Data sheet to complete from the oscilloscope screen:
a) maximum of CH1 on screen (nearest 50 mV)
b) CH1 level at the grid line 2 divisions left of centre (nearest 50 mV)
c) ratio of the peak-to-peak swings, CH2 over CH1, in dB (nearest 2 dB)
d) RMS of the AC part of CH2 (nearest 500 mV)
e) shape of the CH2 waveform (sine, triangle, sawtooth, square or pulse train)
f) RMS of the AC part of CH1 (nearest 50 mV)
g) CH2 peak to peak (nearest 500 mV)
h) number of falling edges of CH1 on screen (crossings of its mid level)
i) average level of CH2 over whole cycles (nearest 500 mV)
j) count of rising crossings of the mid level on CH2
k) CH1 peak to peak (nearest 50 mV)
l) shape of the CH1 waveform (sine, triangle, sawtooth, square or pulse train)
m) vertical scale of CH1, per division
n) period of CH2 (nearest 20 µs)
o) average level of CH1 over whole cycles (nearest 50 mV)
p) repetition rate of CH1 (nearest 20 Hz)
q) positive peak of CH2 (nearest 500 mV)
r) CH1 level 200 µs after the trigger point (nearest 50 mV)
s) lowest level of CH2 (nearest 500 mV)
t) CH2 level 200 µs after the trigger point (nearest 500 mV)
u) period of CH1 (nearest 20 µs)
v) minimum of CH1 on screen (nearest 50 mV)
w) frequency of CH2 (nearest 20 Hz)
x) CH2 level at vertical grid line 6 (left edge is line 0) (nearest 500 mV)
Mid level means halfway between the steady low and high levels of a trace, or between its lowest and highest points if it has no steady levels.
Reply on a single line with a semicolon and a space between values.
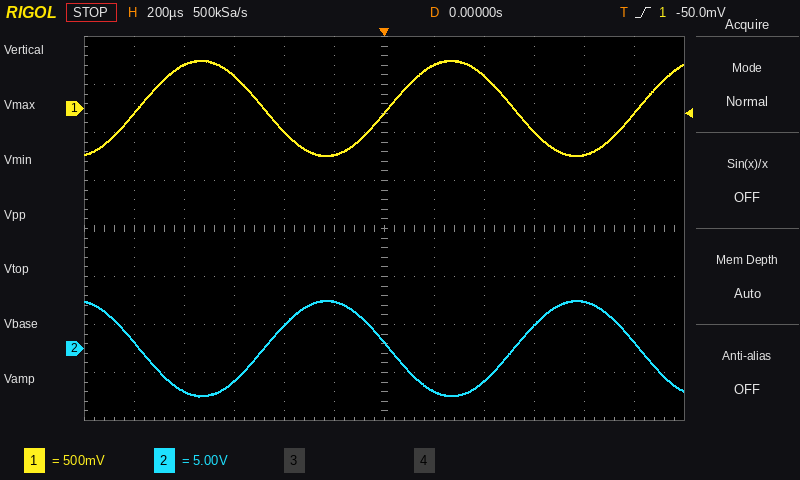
500 mV; -250 mV; 20 dB; 3.5 V; sine; 350 mV; 10.0 V; 2; 0.0 V; 2; 1.00 V; sine; 500 mV; 1.00 ms; 0 mV; 1.00 kHz; 5.0 V; 450 mV; -5.0 V; -4.5 V; 1.00 ms; -500 mV; 1.00 kHz; 500 mV
